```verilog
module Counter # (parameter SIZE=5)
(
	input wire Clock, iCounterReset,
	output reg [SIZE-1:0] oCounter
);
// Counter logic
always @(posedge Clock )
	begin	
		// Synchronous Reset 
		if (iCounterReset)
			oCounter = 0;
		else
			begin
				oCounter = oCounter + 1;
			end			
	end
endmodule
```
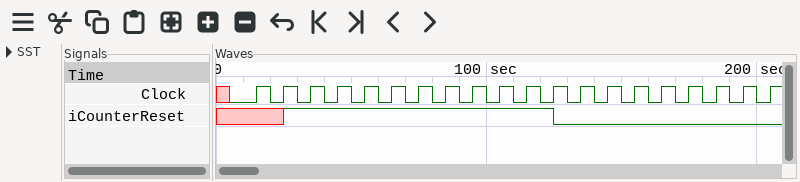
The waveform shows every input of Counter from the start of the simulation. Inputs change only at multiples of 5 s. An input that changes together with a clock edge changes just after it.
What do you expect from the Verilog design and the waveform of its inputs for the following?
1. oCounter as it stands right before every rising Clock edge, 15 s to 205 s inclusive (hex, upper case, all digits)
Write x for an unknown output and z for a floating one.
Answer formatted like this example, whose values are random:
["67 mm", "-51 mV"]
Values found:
["x, x, x, 00, 00, 00, 00, 00, 00, 00, 00, 00, 00, 01, 02, 03, 04, 05, 06, 07"]
